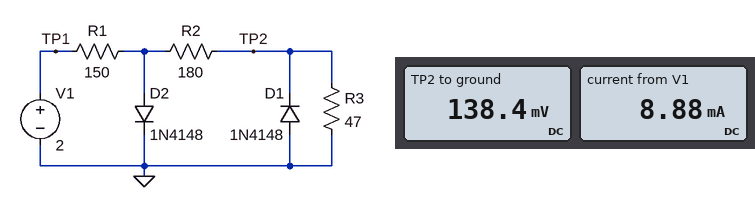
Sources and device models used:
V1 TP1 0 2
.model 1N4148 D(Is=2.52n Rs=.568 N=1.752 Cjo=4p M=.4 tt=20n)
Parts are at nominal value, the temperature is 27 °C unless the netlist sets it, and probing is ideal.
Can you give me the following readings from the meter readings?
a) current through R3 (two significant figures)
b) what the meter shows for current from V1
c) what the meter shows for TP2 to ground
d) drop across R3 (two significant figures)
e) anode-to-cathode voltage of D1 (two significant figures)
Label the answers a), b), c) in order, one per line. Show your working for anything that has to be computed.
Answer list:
a) (138.4 mV) / 47 Ω = 2.9 mA
b) 8.88 mA
c) 138.4 mV
d) 138.4 mV = 140 mV
e) 0 V - 138.4 mV = -140 mV
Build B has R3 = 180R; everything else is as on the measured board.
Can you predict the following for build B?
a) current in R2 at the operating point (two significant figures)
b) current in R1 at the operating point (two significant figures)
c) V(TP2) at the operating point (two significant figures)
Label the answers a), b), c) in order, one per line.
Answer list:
a) 1.9 mA
b) 8.8 mA
c) 340 mV
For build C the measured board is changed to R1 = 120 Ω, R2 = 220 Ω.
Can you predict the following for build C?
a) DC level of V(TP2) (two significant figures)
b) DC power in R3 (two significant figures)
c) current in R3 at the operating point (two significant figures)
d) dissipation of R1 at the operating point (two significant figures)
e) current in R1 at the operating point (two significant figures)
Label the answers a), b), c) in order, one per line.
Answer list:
a) 120 mV
b) 310 µW
c) 2.6 mA
d) 14 mW
e) 11 mA
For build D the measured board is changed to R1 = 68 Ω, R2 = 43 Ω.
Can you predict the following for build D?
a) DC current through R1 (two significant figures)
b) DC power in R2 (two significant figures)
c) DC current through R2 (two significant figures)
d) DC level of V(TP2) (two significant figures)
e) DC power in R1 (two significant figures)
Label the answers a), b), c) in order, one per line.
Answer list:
a) 19 mA
b) 2.6 mW
c) 7.8 mA
d) 370 mV
e) 25 mW
